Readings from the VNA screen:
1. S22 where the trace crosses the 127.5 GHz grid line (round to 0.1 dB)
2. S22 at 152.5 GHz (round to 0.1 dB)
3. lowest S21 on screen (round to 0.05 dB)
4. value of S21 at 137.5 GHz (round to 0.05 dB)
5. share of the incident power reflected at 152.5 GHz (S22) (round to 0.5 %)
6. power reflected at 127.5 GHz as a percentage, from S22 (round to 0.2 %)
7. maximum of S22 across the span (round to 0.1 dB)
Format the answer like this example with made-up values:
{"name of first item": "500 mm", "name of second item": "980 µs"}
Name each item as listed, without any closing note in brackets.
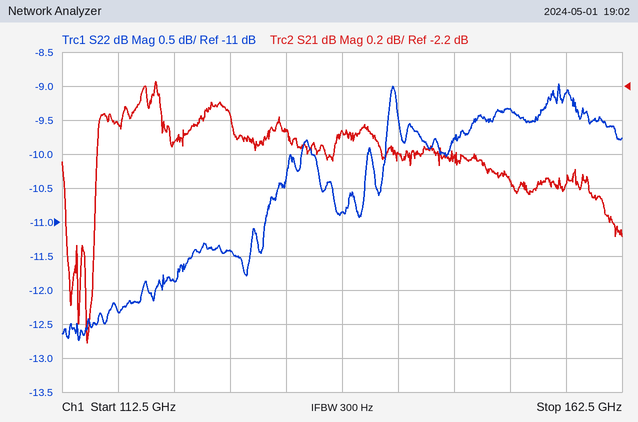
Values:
{"S22 where the trace crosses the 127.5 GHz grid line": "-11.4 dB", "S22 at 152.5 GHz": "-9.3 dB", "lowest S21 on screen": "-3.70 dB", "value of S21 at 137.5 GHz": "-2.45 dB", "share of the incident power reflected at 152.5 GHz (S22)": "11.5 %", "power reflected at 127.5 GHz as a percentage, from S22": "7.2 %", "maximum of S22 across the span": "-9.0 dB"}
